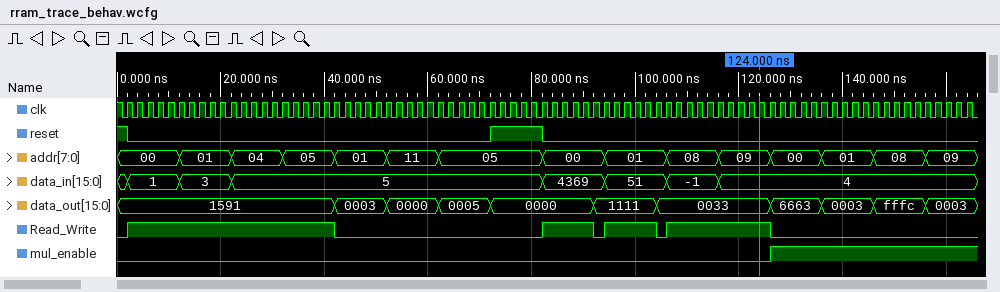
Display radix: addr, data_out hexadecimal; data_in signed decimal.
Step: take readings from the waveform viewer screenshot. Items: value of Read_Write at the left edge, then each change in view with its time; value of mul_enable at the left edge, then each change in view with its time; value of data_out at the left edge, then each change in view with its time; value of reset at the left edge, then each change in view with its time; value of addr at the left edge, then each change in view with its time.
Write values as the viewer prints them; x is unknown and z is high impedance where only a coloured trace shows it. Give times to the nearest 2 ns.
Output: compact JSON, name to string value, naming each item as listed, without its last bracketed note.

{"value of Read_Write at the left edge, then each change in view with its time": "0, 1 at 2 ns, 0 at 42 ns, 1 at 82 ns, 0 at 92 ns, 1 at 94 ns, 0 at 104 ns, 1 at 106 ns, 0 at 126 ns", "value of mul_enable at the left edge, then each change in view with its time": "0, 1 at 126 ns", "value of data_out at the left edge, then each change in view with its time": "1591, 0003 at 42 ns, 0000 at 52 ns, 0005 at 62 ns, 0000 at 72 ns, 1111 at 92 ns, 0033 at 104 ns, 6663 at 126 ns, 0003 at 136 ns, fffc at 146 ns, 0003 at 156 ns", "value of reset at the left edge, then each change in view with its time": "1, 0 at 2 ns, 1 at 72 ns, 0 at 82 ns", "value of addr at the left edge, then each change in view with its time": "00, 01 at 12 ns, 04 at 22 ns, 05 at 32 ns, 01 at 42 ns, 11 at 52 ns, 05 at 62 ns, 00 at 82 ns, 01 at 94 ns, 08 at 106 ns, 09 at 116 ns, 00 at 126 ns, 01 at 136 ns, 08 at 146 ns, 09 at 156 ns"}
